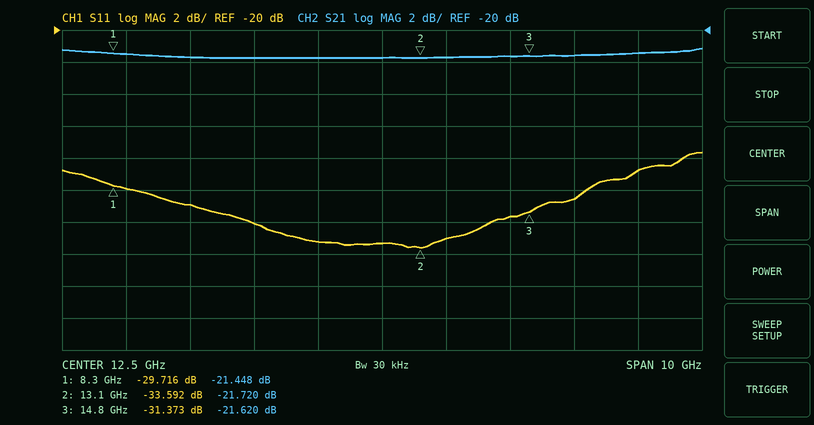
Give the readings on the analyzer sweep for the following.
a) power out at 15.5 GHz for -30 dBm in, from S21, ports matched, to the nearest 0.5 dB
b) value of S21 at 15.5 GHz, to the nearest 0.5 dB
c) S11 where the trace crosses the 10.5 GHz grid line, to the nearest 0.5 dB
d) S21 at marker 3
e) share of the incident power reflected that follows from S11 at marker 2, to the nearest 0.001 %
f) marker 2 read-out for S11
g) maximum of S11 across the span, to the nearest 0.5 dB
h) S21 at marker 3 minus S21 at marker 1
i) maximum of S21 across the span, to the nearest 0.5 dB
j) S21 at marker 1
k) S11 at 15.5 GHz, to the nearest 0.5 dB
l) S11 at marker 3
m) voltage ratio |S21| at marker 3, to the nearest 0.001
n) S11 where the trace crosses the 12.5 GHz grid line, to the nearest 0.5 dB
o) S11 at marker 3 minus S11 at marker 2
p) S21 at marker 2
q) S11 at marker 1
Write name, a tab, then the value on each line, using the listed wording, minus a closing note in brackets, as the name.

power out at 15.5 GHz for -30 dBm in, from S21, ports matched, to the nearest 0.5 dB	-51.5 dBm
value of S21 at 15.5 GHz, to the nearest 0.5 dB	-21.5 dB
S11 where the trace crosses the 10.5 GHz grid line, to the nearest 0.5 dB	-32.0 dB
S21 at marker 3	-21.620 dB
share of the incident power reflected that follows from S11 at marker 2, to the nearest 0.001 %	0.044 %
marker 2 read-out for S11	-33.592 dB
maximum of S11 across the span, to the nearest 0.5 dB	-27.5 dB
S21 at marker 3 minus S21 at marker 1	-0.172 dB
maximum of S21 across the span, to the nearest 0.5 dB	-21.0 dB
S21 at marker 1	-21.448 dB
S11 at 15.5 GHz, to the nearest 0.5 dB	-30.5 dB
S11 at marker 3	-31.373 dB
voltage ratio |S21| at marker 3, to the nearest 0.001	0.083
S11 where the trace crosses the 12.5 GHz grid line, to the nearest 0.5 dB	-33.5 dB
S11 at marker 3 minus S11 at marker 2	2.219 dB
S21 at marker 2	-21.720 dB
S11 at marker 1	-29.716 dB
